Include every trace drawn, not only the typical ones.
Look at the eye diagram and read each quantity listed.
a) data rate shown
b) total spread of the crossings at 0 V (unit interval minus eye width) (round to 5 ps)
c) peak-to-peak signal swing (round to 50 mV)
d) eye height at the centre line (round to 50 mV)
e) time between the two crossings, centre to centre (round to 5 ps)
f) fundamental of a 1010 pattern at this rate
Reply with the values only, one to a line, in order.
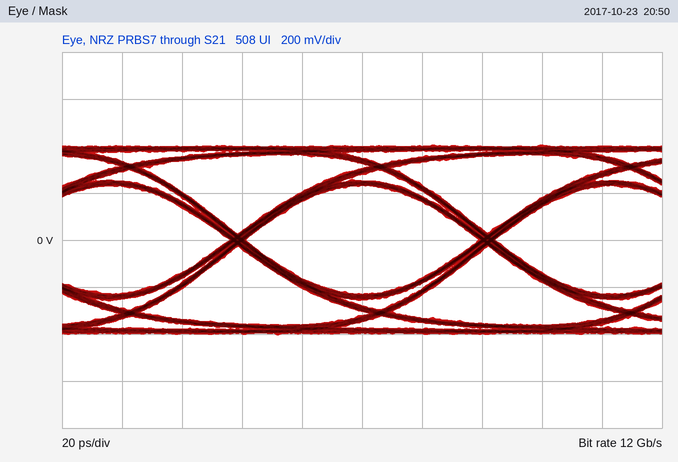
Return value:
12 Gb/s
5 ps
800 mV
450 mV
85 ps
6 GHz
